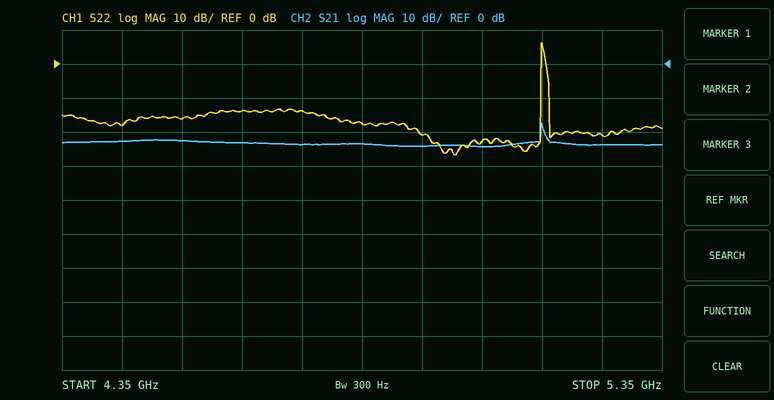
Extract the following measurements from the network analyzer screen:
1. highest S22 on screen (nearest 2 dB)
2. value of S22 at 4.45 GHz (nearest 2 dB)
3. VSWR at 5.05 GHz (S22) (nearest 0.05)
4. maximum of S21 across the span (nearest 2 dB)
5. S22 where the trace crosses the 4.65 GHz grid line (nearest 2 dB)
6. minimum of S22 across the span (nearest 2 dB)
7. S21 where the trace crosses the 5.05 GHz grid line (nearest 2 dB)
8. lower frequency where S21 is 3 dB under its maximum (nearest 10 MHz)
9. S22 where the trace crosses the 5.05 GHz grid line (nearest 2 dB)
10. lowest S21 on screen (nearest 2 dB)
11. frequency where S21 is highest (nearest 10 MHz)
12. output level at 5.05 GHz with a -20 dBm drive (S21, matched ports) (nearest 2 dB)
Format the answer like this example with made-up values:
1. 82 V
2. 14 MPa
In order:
1. 6 dB
2. -18 dB
3. 1.15
4. -18 dB
5. -14 dB
6. -26 dB
7. -24 dB
8. 5.15 GHz
9. -22 dB
10. -24 dB
11. 5.15 GHz
12. -44 dBm
